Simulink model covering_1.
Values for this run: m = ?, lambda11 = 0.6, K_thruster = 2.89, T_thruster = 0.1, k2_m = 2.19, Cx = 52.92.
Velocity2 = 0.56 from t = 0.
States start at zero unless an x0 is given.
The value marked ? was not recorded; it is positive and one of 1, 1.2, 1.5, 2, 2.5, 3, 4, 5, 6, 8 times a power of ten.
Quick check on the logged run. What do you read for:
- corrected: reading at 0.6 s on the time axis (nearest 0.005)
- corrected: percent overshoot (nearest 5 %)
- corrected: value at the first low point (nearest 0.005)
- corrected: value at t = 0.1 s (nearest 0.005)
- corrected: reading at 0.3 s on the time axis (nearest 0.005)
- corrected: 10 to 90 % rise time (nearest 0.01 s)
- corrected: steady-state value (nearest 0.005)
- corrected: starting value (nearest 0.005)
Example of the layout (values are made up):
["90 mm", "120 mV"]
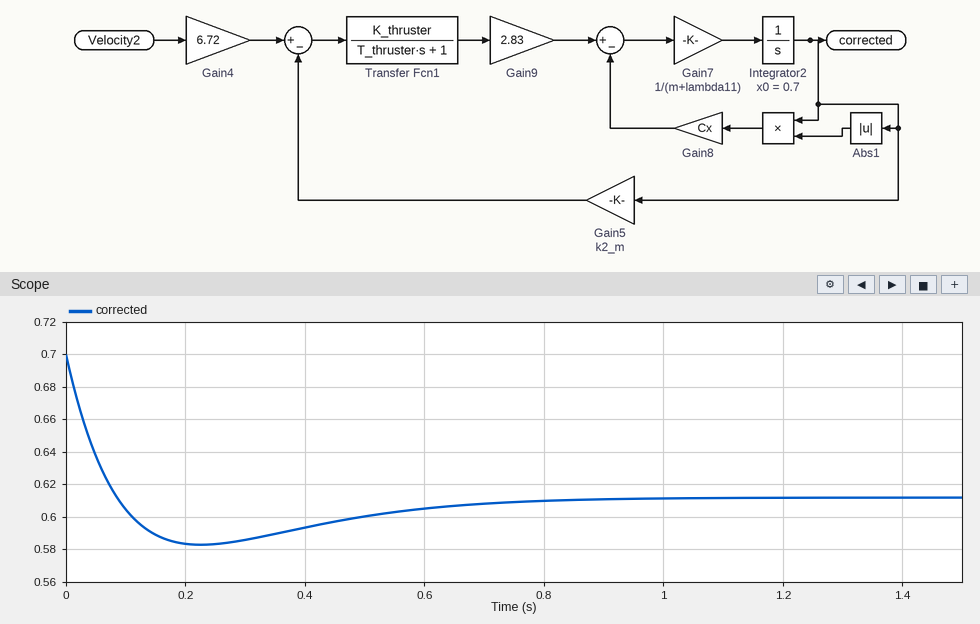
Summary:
["0.605", "35 %", "0.585", "0.605", "0.585", "0.07 s", "0.610", "0.700"]
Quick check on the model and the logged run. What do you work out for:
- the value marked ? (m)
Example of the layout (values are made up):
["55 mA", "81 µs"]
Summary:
["15"]
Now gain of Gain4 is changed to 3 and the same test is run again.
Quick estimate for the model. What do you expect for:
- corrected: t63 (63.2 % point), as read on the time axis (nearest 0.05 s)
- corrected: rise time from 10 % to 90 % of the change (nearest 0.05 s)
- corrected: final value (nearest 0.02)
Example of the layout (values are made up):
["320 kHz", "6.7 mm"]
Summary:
["0.20 s", "0.45 s", "0.36"]
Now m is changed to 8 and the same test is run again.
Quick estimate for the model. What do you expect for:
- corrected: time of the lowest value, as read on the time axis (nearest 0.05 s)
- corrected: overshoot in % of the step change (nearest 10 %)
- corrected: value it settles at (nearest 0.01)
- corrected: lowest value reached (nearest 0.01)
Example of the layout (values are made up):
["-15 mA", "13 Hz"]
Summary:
["0.15 s", "70 %", "0.61", "0.55"]
